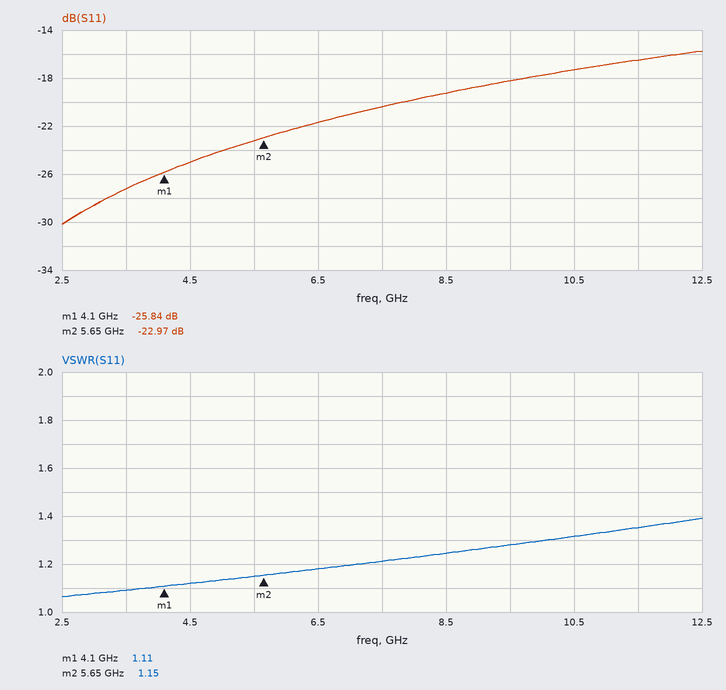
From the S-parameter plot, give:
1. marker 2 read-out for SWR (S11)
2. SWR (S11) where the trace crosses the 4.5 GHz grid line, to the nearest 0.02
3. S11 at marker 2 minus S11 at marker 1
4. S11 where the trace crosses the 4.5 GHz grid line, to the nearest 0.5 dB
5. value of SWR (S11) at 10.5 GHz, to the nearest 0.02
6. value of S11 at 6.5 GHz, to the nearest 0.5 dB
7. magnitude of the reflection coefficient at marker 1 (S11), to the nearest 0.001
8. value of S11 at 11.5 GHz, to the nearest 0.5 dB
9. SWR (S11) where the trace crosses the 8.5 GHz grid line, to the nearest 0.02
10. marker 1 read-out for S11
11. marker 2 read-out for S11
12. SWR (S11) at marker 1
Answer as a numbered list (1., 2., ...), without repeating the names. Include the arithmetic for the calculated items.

1. 1.15
2. 1.12
3. -22.97 − (-25.84) = 2.87 dB
4. -25.0 dB
5. 1.32
6. -21.5 dB
7. 10^(-25.84/20) ≈ 0.051
8. -16.5 dB
9. 1.24
10. -25.84 dB
11. -22.97 dB
12. 1.11
